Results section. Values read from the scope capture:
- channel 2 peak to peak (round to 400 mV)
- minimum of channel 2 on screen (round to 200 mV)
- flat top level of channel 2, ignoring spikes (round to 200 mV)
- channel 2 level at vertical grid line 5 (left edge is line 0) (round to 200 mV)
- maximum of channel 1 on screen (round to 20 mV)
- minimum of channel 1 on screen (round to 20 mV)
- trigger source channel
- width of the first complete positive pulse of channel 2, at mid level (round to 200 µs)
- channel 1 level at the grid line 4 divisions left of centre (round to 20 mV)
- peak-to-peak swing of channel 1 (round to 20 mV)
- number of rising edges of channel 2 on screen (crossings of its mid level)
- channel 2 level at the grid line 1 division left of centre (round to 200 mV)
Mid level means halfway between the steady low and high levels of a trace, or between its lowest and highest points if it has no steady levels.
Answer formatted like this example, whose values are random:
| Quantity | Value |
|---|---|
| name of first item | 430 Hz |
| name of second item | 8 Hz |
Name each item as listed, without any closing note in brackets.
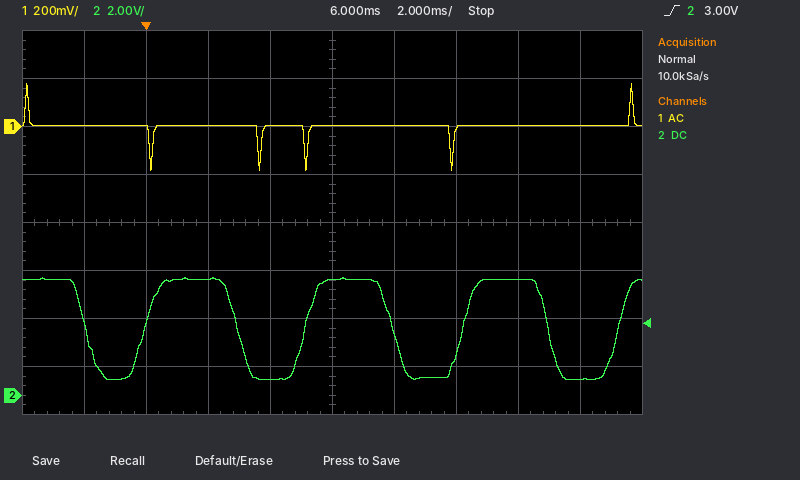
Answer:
| Quantity | Value |
|---|---|
| channel 2 peak to peak | 4.4 V |
| minimum of channel 2 on screen | 600 mV |
| flat top level of channel 2, ignoring spikes | 4.8 V |
| channel 2 level at vertical grid line 5 (left edge is line 0) | 4.8 V |
| maximum of channel 1 on screen | 180 mV |
| minimum of channel 1 on screen | -180 mV |
| trigger source channel | channel 2 |
| width of the first complete positive pulse of channel 2, at mid level | 3.0 ms |
| channel 1 level at the grid line 4 divisions left of centre | 0 mV |
| peak-to-peak swing of channel 1 | 360 mV |
| number of rising edges of channel 2 on screen | 4 |
| channel 2 level at the grid line 1 division left of centre | 600 mV |
